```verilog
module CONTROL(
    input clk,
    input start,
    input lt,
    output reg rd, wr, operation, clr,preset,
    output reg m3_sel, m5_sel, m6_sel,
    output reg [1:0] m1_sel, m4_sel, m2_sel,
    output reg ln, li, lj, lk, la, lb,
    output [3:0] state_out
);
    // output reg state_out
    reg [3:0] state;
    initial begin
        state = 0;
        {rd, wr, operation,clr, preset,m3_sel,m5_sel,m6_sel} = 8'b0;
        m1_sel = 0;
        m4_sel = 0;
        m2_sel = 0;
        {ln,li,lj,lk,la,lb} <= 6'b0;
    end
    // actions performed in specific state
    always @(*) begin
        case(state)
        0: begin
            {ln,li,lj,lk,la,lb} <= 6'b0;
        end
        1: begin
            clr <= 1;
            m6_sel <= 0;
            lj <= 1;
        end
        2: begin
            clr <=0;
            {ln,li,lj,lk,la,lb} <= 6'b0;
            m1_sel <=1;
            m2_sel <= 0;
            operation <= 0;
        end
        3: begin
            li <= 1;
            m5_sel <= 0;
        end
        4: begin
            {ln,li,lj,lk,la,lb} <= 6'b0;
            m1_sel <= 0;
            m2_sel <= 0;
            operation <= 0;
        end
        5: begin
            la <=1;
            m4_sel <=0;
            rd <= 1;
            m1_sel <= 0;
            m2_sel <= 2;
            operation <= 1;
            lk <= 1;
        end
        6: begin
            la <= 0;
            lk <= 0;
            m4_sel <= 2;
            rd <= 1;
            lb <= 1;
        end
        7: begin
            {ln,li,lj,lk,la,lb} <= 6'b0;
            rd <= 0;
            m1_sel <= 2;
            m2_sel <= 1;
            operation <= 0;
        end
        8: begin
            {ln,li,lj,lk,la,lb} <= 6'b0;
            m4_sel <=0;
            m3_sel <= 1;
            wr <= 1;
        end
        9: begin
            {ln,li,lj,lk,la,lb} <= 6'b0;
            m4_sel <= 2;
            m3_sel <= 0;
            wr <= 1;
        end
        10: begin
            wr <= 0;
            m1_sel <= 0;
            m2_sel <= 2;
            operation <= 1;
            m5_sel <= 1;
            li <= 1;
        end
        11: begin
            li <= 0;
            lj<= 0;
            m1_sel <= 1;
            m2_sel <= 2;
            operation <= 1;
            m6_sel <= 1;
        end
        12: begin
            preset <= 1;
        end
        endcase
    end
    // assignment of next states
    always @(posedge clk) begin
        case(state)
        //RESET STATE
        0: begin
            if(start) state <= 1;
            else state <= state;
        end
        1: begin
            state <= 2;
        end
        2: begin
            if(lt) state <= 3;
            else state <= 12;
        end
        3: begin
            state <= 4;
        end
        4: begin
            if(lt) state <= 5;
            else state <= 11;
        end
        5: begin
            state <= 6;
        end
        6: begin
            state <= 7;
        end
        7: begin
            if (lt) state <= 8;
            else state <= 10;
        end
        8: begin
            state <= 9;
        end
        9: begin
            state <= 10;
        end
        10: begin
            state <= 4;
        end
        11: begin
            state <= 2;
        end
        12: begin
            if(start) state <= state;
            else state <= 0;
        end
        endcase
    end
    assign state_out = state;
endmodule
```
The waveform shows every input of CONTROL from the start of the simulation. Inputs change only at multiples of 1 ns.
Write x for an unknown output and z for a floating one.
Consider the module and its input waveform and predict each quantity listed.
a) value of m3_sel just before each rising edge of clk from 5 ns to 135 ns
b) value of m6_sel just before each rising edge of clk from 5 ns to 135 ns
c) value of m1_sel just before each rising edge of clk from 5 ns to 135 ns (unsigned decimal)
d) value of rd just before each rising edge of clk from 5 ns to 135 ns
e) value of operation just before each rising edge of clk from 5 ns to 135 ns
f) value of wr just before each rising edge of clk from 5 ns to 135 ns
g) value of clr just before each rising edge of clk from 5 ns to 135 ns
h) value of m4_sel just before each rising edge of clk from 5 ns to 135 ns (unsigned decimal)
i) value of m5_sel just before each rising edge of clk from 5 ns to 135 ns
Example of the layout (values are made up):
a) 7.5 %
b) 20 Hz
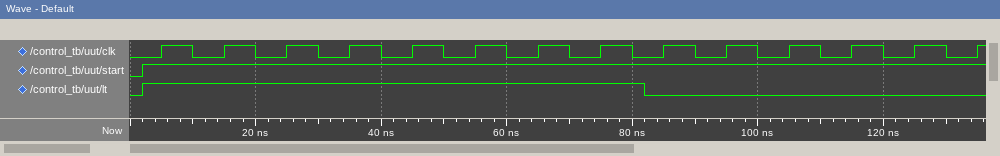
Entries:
a) 0 0 0 0 0 0 0 0 1 0 0 0 0 0
b) 0 0 0 0 0 0 0 0 0 0 0 0 1 1
c) 0, 0, 1, 1, 0, 0, 0, 2, 2, 2, 0, 0, 1, 1
d) 0 0 0 0 0 1 1 0 0 0 0 0 0 0
e) 0 0 0 0 0 1 1 0 0 0 1 0 1 0
f) 0 0 0 0 0 0 0 0 1 1 0 0 0 0
g) 0 1 0 0 0 0 0 0 0 0 0 0 0 0
h) 0, 0, 0, 0, 0, 0, 2, 2, 0, 2, 2, 2, 2, 2
i) 0 0 0 0 0 0 0 0 0 0 1 1 1 1
